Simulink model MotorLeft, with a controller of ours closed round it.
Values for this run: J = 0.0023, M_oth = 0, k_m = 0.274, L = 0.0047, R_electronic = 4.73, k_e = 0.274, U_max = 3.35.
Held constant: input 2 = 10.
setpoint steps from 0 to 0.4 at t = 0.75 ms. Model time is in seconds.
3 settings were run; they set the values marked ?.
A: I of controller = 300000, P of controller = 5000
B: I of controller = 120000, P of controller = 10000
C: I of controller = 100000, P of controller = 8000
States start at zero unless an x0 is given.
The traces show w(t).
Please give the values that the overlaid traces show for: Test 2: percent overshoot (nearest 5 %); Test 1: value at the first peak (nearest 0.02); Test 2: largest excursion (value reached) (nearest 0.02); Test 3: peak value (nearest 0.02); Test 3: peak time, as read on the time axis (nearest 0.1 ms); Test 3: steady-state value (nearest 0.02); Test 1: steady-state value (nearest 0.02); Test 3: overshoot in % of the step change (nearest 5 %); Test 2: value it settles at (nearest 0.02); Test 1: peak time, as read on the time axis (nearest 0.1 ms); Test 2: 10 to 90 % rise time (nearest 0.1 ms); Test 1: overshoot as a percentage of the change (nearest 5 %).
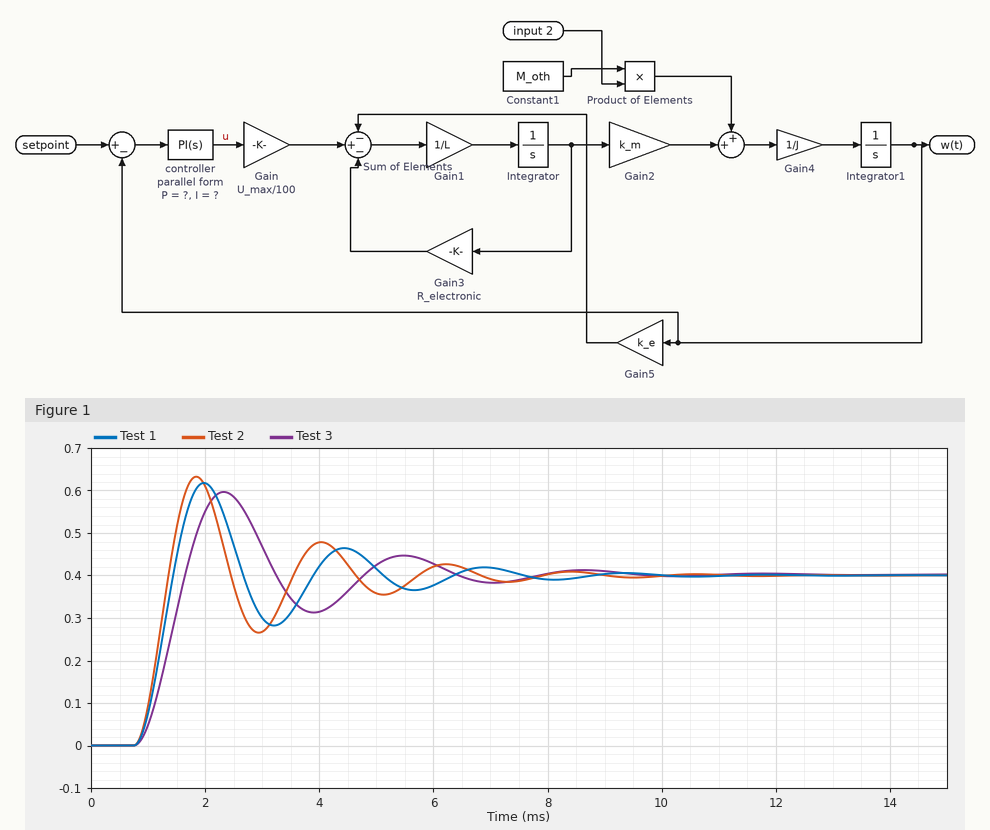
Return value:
60 %
0.62
0.64
0.60
2.3 ms
0.40
0.40
50 %
0.40
2.0 ms
0.4 ms
55 %
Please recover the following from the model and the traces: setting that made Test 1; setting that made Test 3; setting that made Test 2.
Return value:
C
A
B
